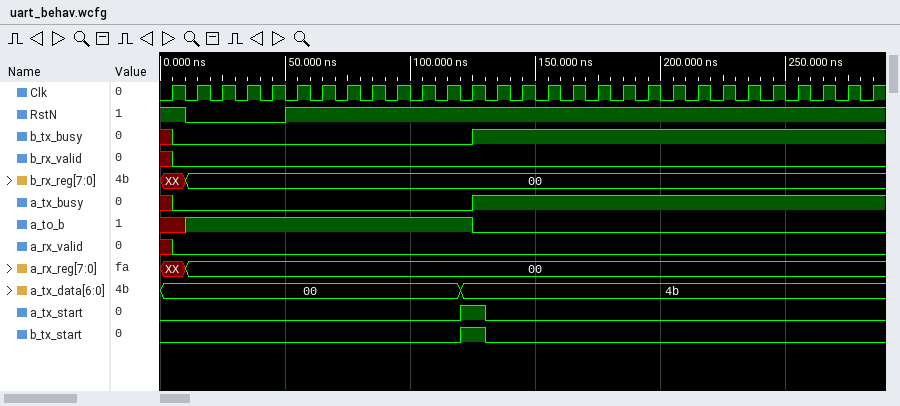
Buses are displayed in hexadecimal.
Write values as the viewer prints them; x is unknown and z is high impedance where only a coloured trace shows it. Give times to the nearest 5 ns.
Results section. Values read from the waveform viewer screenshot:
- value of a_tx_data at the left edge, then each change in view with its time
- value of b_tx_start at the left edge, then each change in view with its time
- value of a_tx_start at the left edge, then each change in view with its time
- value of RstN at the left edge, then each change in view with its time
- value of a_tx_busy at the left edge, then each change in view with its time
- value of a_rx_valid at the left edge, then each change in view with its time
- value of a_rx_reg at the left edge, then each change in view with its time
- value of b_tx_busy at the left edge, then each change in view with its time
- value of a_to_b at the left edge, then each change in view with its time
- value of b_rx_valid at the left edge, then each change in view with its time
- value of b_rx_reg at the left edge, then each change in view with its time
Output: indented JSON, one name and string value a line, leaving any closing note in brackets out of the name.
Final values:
{
  "value of a_tx_data at the left edge, then each change in view with its time": "00, 4b at 120 ns",
  "value of b_tx_start at the left edge, then each change in view with its time": "0, 1 at 120 ns, 0 at 130 ns",
  "value of a_tx_start at the left edge, then each change in view with its time": "0, 1 at 120 ns, 0 at 130 ns",
  "value of RstN at the left edge, then each change in view with its time": "1, 0 at 10 ns, 1 at 50 ns",
  "value of a_tx_busy at the left edge, then each change in view with its time": "x, 0 at 5 ns, 1 at 125 ns",
  "value of a_rx_valid at the left edge, then each change in view with its time": "x, 0 at 5 ns",
  "value of a_rx_reg at the left edge, then each change in view with its time": "XX, 00 at 10 ns",
  "value of b_tx_busy at the left edge, then each change in view with its time": "x, 0 at 5 ns, 1 at 125 ns",
  "value of a_to_b at the left edge, then each change in view with its time": "x, 1 at 10 ns, 0 at 125 ns",
  "value of b_rx_valid at the left edge, then each change in view with its time": "x, 0 at 5 ns",
  "value of b_rx_reg at the left edge, then each change in view with its time": "XX, 00 at 10 ns"
}
